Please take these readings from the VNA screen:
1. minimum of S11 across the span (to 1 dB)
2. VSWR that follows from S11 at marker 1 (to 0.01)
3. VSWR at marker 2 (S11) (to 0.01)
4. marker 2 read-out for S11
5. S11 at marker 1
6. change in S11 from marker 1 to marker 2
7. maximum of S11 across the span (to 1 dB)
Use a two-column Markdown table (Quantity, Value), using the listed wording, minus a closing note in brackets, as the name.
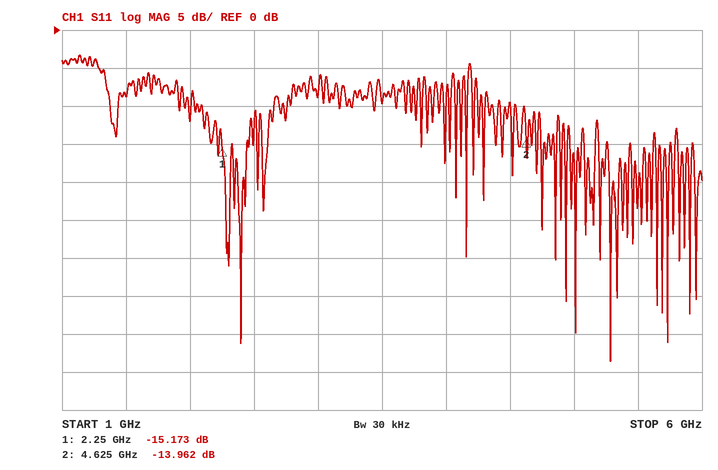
| Quantity | Value |
|---|---|
| minimum of S11 across the span | -44 dB |
| VSWR that follows from S11 at marker 1 | 1.42 |
| VSWR at marker 2 (S11) | 1.50 |
| marker 2 read-out for S11 | -13.962 dB |
| S11 at marker 1 | -15.173 dB |
| change in S11 from marker 1 to marker 2 | 1.211 dB |
| maximum of S11 across the span | -3 dB |
